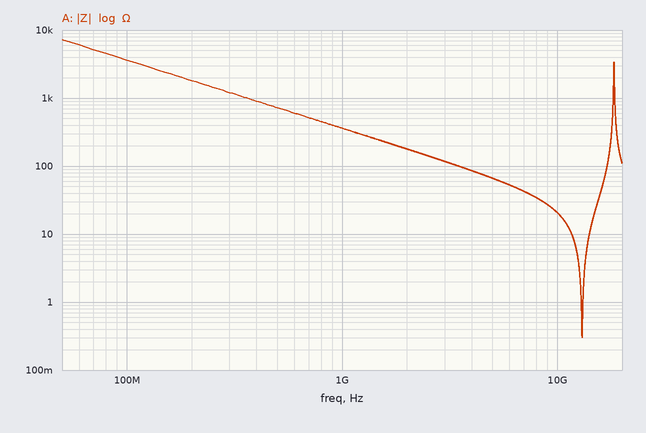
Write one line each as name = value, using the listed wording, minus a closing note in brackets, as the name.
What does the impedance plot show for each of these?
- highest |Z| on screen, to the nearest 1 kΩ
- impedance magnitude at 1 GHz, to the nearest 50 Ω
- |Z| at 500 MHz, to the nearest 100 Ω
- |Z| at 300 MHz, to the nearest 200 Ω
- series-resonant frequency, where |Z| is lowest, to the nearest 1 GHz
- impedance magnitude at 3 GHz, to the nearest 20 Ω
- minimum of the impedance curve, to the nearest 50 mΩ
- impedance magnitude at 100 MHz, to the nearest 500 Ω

highest |Z| on screen, to the nearest 1 kΩ = 7 kΩ
impedance magnitude at 1 GHz, to the nearest 50 Ω = 350 Ω
|Z| at 500 MHz, to the nearest 100 Ω = 700 Ω
|Z| at 300 MHz, to the nearest 200 Ω = 1.2 kΩ
series-resonant frequency, where |Z| is lowest, to the nearest 1 GHz = 13 GHz
impedance magnitude at 3 GHz, to the nearest 20 Ω = 120 Ω
minimum of the impedance curve, to the nearest 50 mΩ = 300 mΩ
impedance magnitude at 100 MHz, to the nearest 500 Ω = 3.5 kΩ
